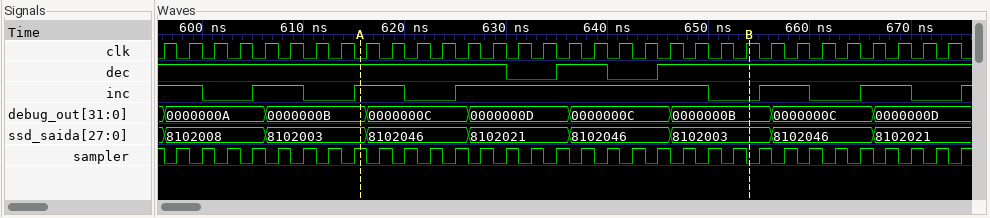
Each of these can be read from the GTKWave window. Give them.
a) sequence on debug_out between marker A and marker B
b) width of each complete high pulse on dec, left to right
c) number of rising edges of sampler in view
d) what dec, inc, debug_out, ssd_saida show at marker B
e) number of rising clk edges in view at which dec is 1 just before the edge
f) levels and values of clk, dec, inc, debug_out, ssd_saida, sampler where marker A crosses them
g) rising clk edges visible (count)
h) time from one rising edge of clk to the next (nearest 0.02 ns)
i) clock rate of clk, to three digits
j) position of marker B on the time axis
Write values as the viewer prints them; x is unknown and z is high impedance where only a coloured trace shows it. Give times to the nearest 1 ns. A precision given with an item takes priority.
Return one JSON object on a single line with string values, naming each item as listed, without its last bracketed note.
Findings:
{"sequence on debug_out between marker A and marker B": "0000000B, 0000000C, 0000000D, 0000000C, 0000000B", "width of each complete high pulse on dec, left to right": "5 ns", "number of rising edges of sampler in view": "32", "what dec, inc, debug_out, ssd_saida show at marker B": "dec=1, inc=0, debug_out=0000000B, ssd_saida=8102003", "number of rising clk edges in view at which dec is 1 just before the edge": "28", "levels and values of clk, dec, inc, debug_out, ssd_saida, sampler where marker A crosses them": "clk=0, dec=1, inc=1, debug_out=0000000B, ssd_saida=8102003, sampler=1", "rising clk edges visible": "32", "time from one rising edge of clk to the next": "2.5 ns", "clock rate of clk, to three digits": "400 MHz", "position of marker B on the time axis": "654 ns"}
